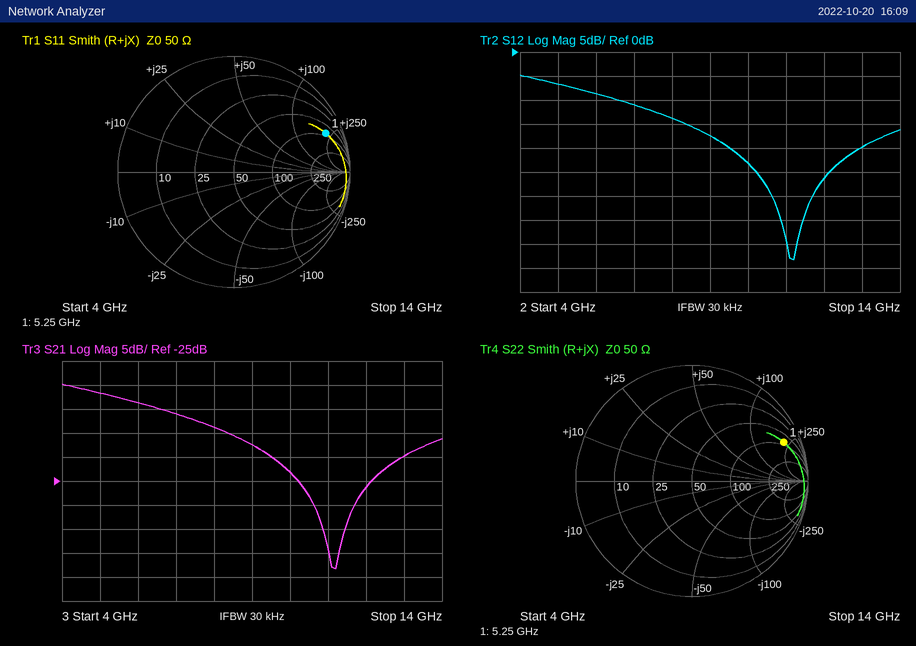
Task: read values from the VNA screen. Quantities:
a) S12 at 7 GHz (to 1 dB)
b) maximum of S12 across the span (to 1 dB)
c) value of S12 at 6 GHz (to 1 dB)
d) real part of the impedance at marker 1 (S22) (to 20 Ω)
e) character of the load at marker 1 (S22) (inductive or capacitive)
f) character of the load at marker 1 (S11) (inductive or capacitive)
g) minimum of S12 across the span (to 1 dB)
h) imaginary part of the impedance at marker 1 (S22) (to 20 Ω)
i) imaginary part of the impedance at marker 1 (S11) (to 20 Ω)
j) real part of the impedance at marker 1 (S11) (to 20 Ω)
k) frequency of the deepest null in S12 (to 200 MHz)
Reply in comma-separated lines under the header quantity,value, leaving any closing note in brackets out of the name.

quantity,value
S12 at 7 GHz,-11 dB
maximum of S12 across the span,-5 dB
value of S12 at 6 GHz,-9 dB
real part of the impedance at marker 1 (S22),80 Ω
character of the load at marker 1 (S22),inductive
character of the load at marker 1 (S11),inductive
minimum of S12 across the span,-43 dB
imaginary part of the impedance at marker 1 (S22),+220 Ω
imaginary part of the impedance at marker 1 (S11),+220 Ω
real part of the impedance at marker 1 (S11),80 Ω
frequency of the deepest null in S12,11.2 GHz
